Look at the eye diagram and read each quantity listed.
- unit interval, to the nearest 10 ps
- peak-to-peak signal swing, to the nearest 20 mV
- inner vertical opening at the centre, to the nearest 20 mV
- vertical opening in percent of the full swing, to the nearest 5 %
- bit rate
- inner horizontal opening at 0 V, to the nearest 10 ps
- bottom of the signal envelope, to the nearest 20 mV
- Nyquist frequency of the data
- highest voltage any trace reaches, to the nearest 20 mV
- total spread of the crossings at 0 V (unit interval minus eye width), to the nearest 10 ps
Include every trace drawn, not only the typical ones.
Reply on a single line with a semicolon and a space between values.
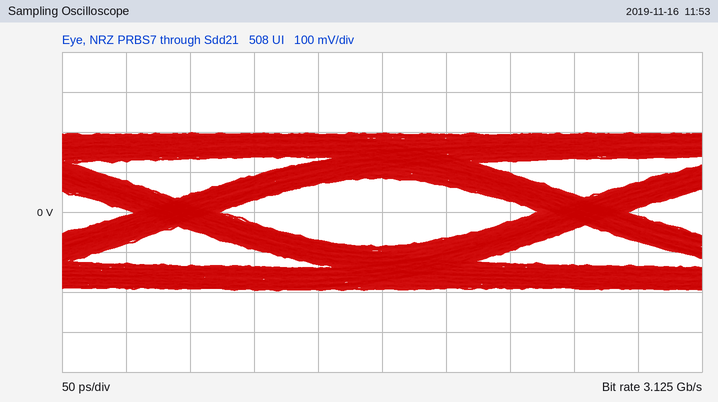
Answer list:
320 ps; 400 mV; 180 mV; 45 %; 3.125 Gb/s; 250 ps; -200 mV; 1.5625 GHz; 200 mV; 70 ps
